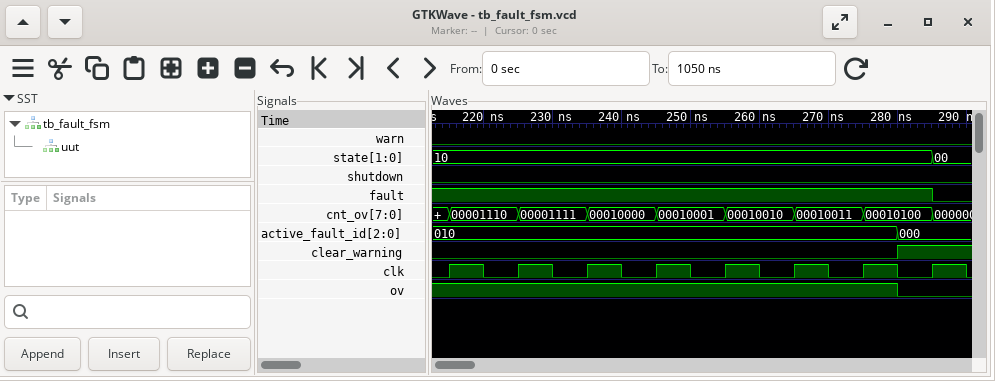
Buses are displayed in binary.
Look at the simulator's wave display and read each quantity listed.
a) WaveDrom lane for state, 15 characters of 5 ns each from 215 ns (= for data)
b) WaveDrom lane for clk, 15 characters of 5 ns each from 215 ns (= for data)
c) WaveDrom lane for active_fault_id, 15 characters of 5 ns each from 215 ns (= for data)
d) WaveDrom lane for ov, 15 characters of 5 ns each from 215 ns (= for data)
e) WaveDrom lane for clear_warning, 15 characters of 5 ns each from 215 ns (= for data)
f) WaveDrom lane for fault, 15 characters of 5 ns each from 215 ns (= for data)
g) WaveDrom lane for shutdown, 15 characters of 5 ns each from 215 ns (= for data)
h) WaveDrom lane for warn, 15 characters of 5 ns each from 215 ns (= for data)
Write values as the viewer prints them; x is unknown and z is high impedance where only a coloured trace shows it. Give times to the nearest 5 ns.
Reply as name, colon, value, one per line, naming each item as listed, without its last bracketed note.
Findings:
WaveDrom lane for state, 15 characters of 5 ns each from 215 ns: {name: 'state', wave: '=.............=', data: '10 00'}
WaveDrom lane for clk, 15 characters of 5 ns each from 215 ns: {name: 'clk', wave: '101010101010101'}
WaveDrom lane for active_fault_id, 15 characters of 5 ns each from 215 ns: {name: 'active_fault_id', wave: '=............=.', data: '010 000'}
WaveDrom lane for ov, 15 characters of 5 ns each from 215 ns: {name: 'ov', wave: '1............0.'}
WaveDrom lane for clear_warning, 15 characters of 5 ns each from 215 ns: {name: 'clear_warning', wave: '0............1.'}
WaveDrom lane for fault, 15 characters of 5 ns each from 215 ns: {name: 'fault', wave: '1.............0'}
WaveDrom lane for shutdown, 15 characters of 5 ns each from 215 ns: {name: 'shutdown', wave: '0..............'}
WaveDrom lane for warn, 15 characters of 5 ns each from 215 ns: {name: 'warn', wave: '0..............'}
